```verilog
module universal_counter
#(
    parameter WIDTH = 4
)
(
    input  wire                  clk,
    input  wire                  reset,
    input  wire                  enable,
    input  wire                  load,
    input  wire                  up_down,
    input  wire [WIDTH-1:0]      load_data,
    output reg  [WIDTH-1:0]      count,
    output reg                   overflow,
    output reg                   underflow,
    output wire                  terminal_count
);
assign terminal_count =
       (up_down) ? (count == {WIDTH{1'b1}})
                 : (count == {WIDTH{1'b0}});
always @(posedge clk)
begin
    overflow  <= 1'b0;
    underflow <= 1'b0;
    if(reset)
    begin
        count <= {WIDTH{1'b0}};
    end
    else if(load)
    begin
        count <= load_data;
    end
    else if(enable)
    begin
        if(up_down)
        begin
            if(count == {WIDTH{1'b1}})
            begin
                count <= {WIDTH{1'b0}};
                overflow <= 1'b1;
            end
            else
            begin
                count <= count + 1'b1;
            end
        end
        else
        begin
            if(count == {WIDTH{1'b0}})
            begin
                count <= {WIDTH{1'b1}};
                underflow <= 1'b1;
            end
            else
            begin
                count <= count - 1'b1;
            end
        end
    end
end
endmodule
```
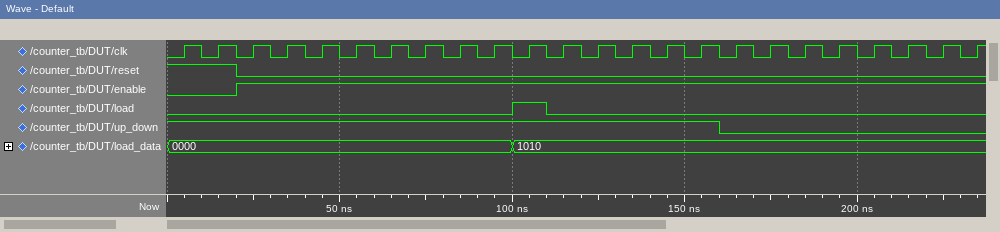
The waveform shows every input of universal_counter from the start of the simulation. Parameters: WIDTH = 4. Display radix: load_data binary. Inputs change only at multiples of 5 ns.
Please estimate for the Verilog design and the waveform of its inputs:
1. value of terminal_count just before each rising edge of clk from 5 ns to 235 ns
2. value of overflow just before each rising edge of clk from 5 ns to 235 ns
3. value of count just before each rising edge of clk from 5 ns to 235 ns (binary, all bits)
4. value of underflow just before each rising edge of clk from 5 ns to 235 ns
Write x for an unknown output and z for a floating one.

x 0 0 0 0 0 0 0 0 0 0 0 0 0 0 0 0 0 0 0 0 0 0 0
x 0 0 0 0 0 0 0 0 0 0 0 0 0 0 0 0 0 0 0 0 0 0 0
x, 0000, 0000, 0001, 0010, 0011, 0100, 0101, 0110, 0111, 1000, 1010, 1011, 1100, 1101, 1110, 1111, 1110, 1101, 1100, 1011, 1010, 1001, 1000
x 0 0 0 0 0 0 0 0 0 0 0 0 0 0 0 0 0 0 0 0 0 0 0
